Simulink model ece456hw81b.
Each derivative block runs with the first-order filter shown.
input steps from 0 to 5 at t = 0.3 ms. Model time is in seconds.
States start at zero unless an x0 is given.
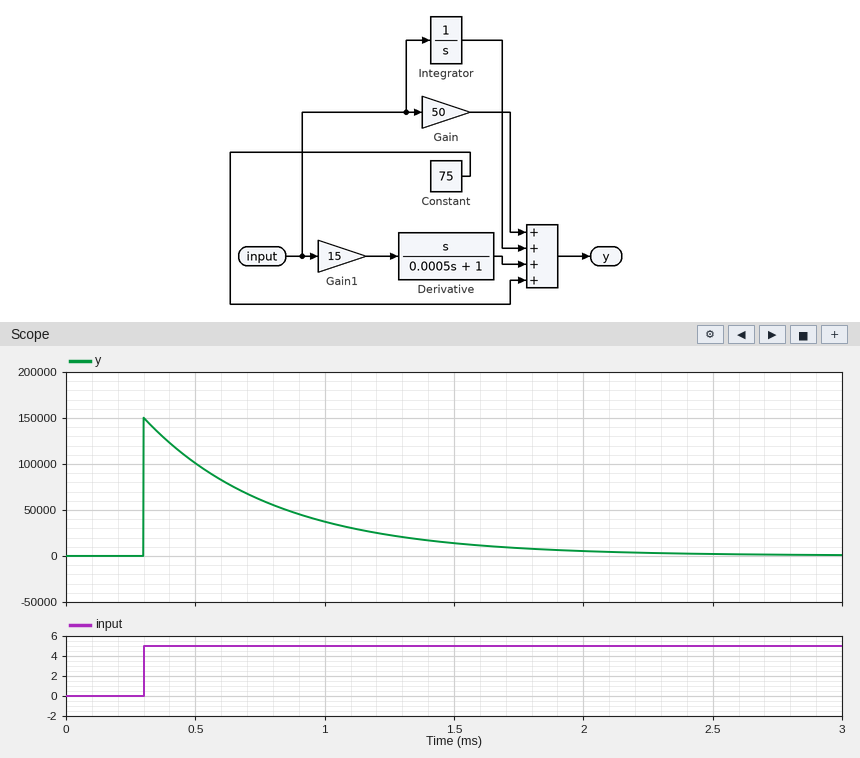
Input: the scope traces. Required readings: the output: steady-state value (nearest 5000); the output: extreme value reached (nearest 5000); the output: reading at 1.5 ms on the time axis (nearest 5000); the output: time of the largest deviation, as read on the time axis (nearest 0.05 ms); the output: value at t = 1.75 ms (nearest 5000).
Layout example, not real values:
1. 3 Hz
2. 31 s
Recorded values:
1. 0
2. 150000
3. 15000
4. 0.30 ms
5. 10000
